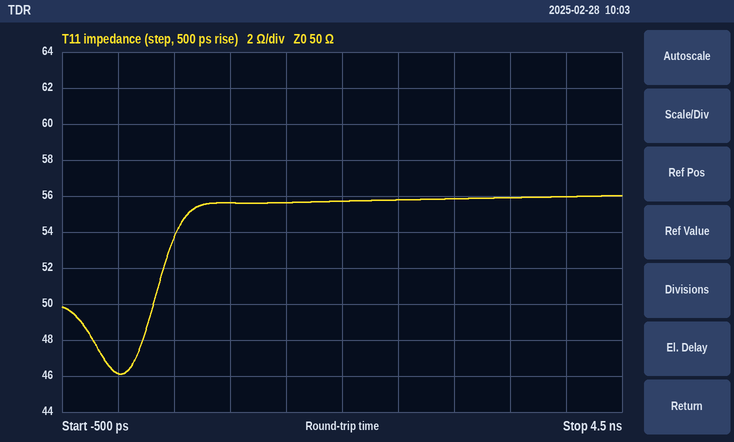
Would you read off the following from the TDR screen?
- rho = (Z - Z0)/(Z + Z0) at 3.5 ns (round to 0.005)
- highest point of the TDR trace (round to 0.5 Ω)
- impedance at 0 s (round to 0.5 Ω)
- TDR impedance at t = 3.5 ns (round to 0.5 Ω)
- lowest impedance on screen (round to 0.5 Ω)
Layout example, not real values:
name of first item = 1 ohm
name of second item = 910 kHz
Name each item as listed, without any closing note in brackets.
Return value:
rho = (Z - Z0)/(Z + Z0) at 3.5 ns = +0.055
highest point of the TDR trace = 56.0 Ω
impedance at 0 s = 46.0 Ω
TDR impedance at t = 3.5 ns = 56.0 Ω
lowest impedance on screen = 46.0 Ω
